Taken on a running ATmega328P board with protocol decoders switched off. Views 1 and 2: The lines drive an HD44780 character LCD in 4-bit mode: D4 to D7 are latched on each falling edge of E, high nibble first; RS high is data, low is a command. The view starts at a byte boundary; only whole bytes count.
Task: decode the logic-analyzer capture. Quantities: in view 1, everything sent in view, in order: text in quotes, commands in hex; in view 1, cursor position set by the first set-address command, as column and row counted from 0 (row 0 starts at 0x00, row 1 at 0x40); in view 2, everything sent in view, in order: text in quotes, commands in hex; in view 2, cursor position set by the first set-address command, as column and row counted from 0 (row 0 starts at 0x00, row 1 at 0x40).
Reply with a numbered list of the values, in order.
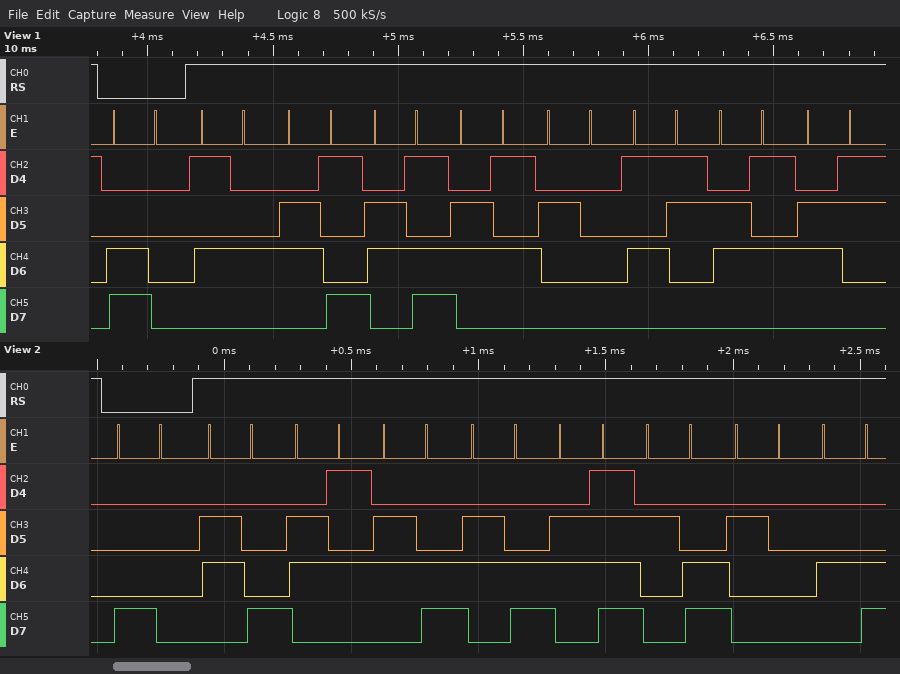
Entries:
1. 0xC0 "Time Sec"
2. column 0, row 1
3. 0x80 "hello, L"
4. column 0, row 0
